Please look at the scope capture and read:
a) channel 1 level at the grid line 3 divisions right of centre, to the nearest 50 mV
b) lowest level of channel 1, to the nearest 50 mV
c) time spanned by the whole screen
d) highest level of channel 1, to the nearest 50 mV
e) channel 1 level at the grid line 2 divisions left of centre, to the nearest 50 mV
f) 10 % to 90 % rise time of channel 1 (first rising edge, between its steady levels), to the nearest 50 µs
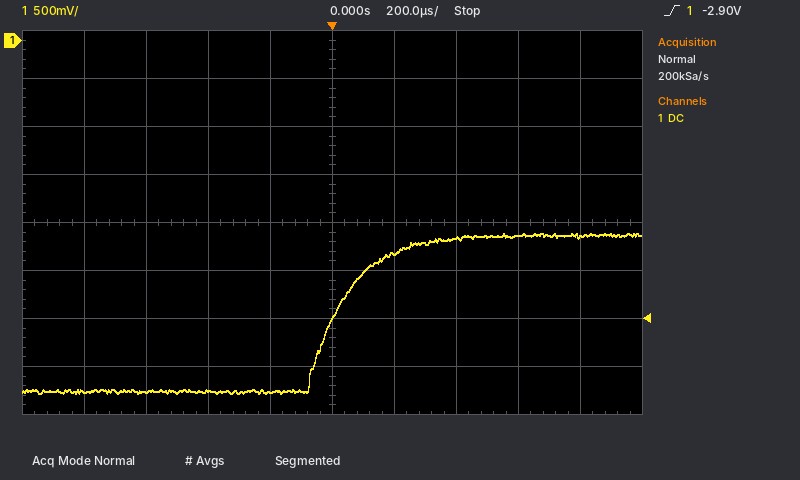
-2.05 V
-3.70 V
2 ms
-2.00 V
-3.65 V
300 µs
